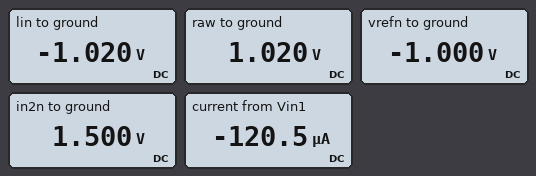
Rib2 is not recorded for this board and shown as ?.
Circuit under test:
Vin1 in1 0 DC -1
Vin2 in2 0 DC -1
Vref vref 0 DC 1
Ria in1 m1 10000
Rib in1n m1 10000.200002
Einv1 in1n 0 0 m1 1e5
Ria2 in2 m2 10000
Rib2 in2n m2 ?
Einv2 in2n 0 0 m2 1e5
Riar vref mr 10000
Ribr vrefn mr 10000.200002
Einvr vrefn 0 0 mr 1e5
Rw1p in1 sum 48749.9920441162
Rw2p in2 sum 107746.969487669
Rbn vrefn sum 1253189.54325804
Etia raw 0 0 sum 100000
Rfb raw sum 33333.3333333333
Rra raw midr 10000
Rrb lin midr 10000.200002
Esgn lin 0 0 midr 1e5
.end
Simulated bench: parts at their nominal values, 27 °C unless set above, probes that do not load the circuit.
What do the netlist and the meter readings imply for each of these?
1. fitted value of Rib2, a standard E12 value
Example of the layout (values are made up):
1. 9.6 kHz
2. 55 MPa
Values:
1. 15 kΩ
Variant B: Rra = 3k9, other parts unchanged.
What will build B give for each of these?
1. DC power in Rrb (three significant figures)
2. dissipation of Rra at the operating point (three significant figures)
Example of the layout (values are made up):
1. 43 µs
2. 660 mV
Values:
1. 684 µW
2. 267 µW
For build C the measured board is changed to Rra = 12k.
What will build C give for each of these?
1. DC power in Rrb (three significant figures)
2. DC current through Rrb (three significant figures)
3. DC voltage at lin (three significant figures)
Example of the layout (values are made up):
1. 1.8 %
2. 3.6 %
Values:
1. 72.2 µW
2. 85.0 µA
3. -850 mV
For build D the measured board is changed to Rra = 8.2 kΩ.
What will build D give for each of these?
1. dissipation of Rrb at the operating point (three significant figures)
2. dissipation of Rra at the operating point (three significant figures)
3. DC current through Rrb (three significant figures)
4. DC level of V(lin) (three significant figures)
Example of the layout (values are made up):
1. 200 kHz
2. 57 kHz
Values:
1. 155 µW
2. 127 µW
3. 124 µA
4. -1.24 V
